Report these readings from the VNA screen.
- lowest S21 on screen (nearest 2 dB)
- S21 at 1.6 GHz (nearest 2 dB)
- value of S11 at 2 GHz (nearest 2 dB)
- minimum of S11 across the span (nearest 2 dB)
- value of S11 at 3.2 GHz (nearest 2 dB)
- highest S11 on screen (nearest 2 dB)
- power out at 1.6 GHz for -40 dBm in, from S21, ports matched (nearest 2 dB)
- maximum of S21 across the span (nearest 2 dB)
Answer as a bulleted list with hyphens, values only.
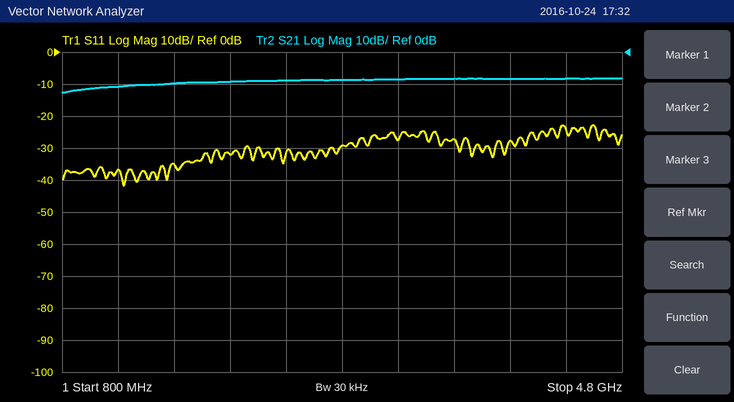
- -12 dB
- -10 dB
- -32 dB
- -42 dB
- -28 dB
- -22 dB
- -50 dBm
- -8 dB
